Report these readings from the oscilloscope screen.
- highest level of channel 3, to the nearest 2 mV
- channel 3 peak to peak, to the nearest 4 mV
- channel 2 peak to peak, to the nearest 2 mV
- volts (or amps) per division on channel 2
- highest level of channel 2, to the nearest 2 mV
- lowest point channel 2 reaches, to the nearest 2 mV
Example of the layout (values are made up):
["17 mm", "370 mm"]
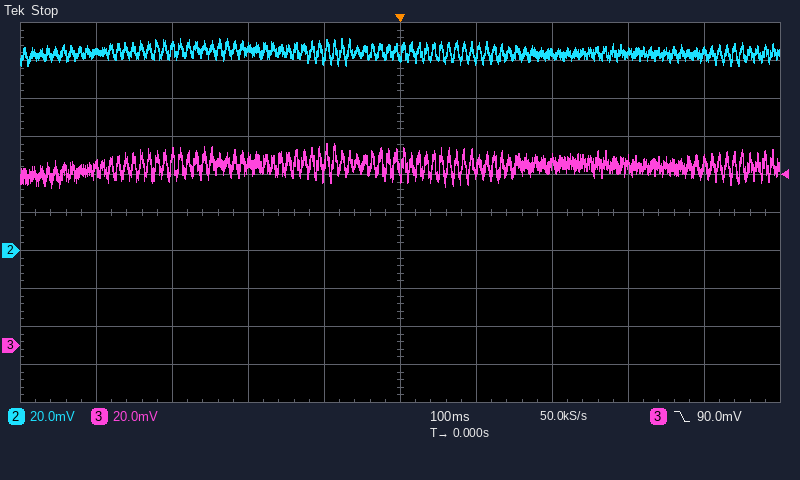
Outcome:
["106 mV", "24 mV", "14 mV", "20 mV", "112 mV", "98 mV"]
